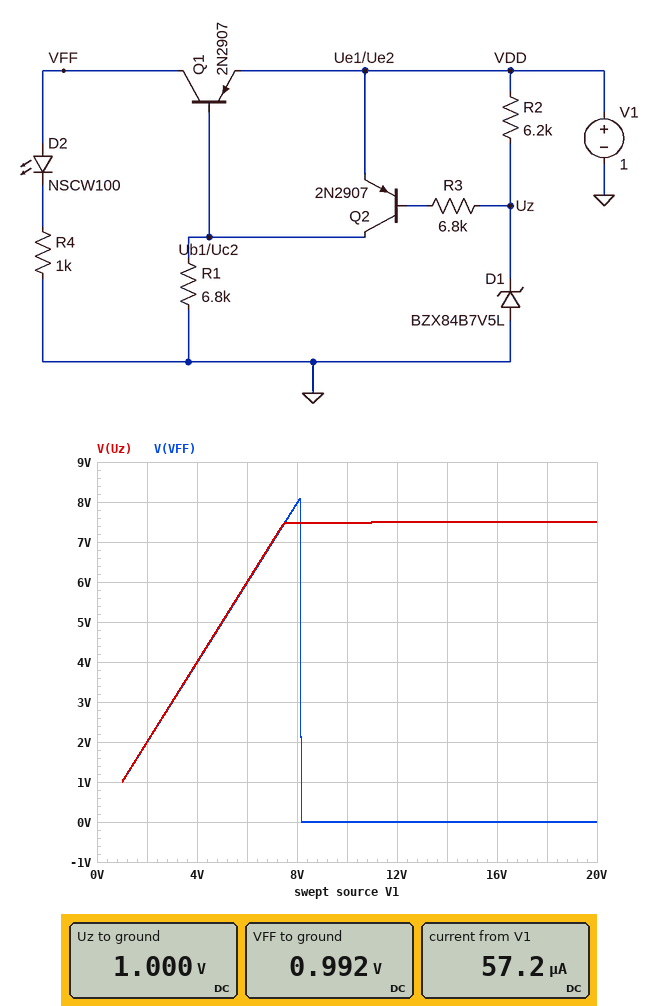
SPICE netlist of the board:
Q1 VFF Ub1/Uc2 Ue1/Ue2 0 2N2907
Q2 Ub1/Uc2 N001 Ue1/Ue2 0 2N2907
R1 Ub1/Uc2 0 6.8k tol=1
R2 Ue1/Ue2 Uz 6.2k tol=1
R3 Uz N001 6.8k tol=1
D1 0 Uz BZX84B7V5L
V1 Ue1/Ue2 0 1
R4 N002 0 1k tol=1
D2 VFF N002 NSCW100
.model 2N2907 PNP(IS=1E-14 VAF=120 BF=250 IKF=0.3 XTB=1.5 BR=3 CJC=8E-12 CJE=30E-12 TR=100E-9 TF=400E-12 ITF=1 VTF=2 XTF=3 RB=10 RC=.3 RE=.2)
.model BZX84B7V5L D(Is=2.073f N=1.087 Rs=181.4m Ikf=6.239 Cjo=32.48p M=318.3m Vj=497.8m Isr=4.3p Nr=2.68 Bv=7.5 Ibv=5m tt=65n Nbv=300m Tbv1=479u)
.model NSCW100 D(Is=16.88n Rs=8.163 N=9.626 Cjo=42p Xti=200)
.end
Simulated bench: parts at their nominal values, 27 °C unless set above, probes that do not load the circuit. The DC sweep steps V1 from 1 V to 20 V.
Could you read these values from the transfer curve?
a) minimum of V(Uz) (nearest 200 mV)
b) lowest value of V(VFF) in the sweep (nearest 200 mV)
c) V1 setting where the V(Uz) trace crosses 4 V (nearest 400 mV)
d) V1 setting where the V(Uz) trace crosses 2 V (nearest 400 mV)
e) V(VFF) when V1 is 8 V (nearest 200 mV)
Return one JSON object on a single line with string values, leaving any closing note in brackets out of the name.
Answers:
{"minimum of V(Uz)": "1.0 V", "lowest value of V(VFF) in the sweep": "0 V", "V1 setting where the V(Uz) trace crosses 4 V": "4.0 V", "V1 setting where the V(Uz) trace crosses 2 V": "2.0 V", "V(VFF) when V1 is 8 V": "8.0 V"}
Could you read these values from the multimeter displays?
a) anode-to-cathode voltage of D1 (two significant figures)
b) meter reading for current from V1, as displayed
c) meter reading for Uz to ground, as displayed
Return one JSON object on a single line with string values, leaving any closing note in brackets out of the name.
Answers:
{"anode-to-cathode voltage of D1": "-1.0 V", "meter reading for current from V1, as displayed": "57.2 µA", "meter reading for Uz to ground, as displayed": "1.000 V"}
